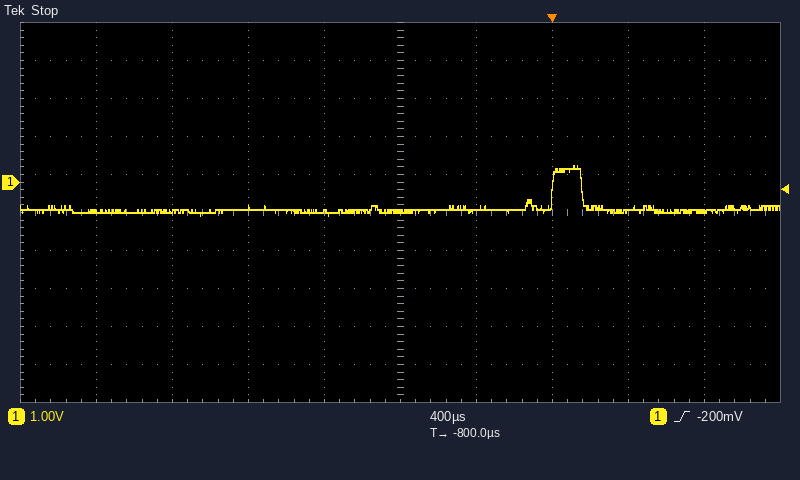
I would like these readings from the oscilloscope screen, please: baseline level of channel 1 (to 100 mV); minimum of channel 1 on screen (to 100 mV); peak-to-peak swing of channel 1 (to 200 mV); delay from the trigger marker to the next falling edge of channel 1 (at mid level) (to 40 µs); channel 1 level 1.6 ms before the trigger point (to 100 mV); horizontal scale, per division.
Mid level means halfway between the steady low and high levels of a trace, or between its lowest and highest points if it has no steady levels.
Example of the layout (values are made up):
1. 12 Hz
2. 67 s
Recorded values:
1. -700 mV
2. -900 mV
3. 1.4 V
4. 160 µs
5. -700 mV
6. 400 µs
